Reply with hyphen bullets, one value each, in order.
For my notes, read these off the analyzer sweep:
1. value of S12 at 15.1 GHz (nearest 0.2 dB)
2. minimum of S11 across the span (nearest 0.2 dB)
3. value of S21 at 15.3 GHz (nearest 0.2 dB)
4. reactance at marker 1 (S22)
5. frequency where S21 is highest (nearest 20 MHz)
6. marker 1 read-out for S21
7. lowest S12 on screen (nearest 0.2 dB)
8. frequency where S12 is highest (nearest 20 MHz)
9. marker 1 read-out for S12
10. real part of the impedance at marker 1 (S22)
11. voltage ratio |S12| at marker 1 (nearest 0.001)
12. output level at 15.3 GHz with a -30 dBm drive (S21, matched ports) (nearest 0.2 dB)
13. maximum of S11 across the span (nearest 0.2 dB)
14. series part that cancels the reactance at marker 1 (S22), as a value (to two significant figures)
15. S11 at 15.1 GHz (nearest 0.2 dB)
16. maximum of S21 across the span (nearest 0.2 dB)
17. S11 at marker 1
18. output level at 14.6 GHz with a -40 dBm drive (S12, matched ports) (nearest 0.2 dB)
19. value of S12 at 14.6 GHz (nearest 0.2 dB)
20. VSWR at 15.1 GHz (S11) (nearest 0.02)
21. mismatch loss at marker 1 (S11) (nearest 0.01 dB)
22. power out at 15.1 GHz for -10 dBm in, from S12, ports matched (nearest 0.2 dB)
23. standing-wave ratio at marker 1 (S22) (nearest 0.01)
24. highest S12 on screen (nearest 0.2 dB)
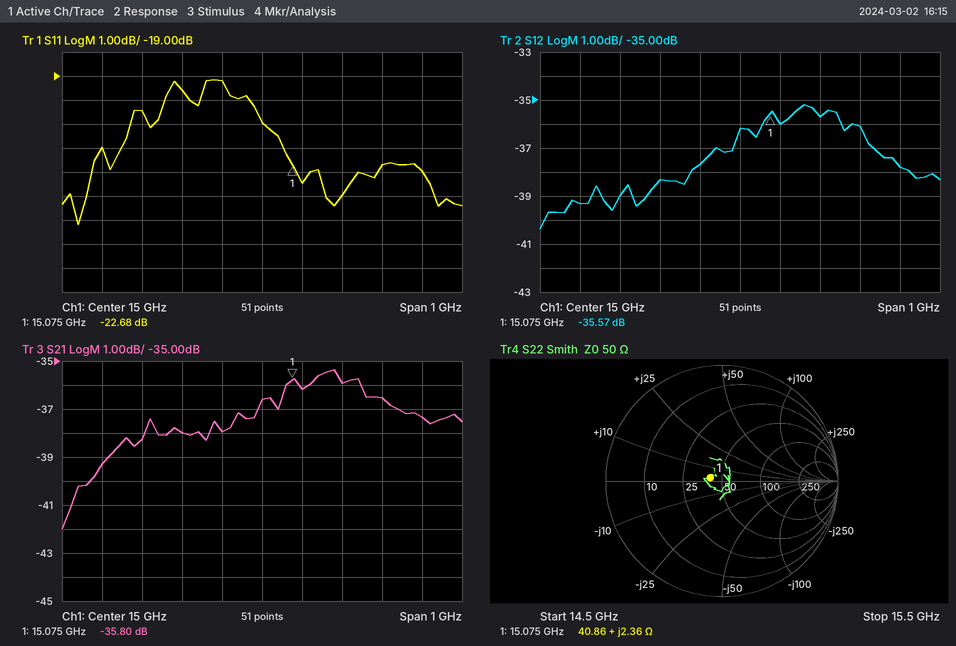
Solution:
- -36.0 dB
- -25.2 dB
- -36.6 dB
- +2.36 Ω
- 15.18 GHz
- -35.80 dB
- -40.4 dB
- 15.16 GHz
- -35.57 dB
- 40.86 Ω
- 0.017
- -66.6 dBm
- -19.2 dB
- 4.5 pF
- -23.4 dB
- -35.4 dB
- -22.68 dB
- -79.4 dBm
- -39.4 dB
- 1.14
- 0.02 dB
- -46.0 dBm
- 1.23
- -35.2 dB
